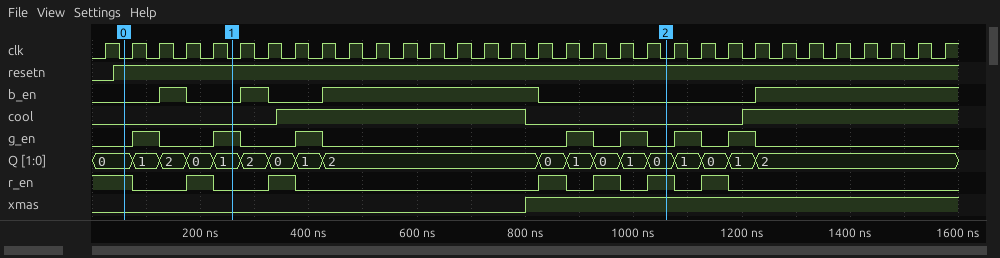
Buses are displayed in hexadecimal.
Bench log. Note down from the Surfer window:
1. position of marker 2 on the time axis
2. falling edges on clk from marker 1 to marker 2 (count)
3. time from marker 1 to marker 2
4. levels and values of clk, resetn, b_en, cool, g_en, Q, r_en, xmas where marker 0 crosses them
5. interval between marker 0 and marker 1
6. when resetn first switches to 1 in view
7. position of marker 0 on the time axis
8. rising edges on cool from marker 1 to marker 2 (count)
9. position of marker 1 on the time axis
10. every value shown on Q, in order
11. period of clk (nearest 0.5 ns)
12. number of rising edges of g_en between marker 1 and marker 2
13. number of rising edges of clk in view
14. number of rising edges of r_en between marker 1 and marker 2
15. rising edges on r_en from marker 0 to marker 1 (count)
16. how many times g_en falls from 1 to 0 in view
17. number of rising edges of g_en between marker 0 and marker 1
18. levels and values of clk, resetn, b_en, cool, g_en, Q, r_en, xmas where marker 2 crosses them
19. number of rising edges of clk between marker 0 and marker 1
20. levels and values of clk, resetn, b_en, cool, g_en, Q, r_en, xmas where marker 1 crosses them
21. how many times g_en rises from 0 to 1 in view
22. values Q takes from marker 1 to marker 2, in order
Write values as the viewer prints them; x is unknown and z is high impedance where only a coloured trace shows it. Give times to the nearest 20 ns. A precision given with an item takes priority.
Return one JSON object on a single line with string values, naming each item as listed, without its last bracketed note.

{"position of marker 2 on the time axis": "1060 ns", "falling edges on clk from marker 1 to marker 2": "16", "time from marker 1 to marker 2": "800 ns", "levels and values of clk, resetn, b_en, cool, g_en, Q, r_en, xmas where marker 0 crosses them": "clk=0, resetn=1, b_en=0, cool=0, g_en=0, Q=0, r_en=1, xmas=0", "interval between marker 0 and marker 1": "200 ns", "when resetn first switches to 1 in view": "40 ns", "position of marker 0 on the time axis": "60 ns", "rising edges on cool from marker 1 to marker 2": "1", "position of marker 1 on the time axis": "260 ns", "every value shown on Q, in order": "0, 1, 2, 0, 1, 2, 0, 1, 2, 0, 1, 0, 1, 0, 1, 0, 1, 2", "period of clk": "50 ns", "number of rising edges of g_en between marker 1 and marker 2": "3", "number of rising edges of clk in view": "32", "number of rising edges of r_en between marker 1 and marker 2": "4", "rising edges on r_en from marker 0 to marker 1": "1", "how many times g_en falls from 1 to 0 in view": "7", "number of rising edges of g_en between marker 0 and marker 1": "2", "levels and values of clk, resetn, b_en, cool, g_en, Q, r_en, xmas where marker 2 crosses them": "clk=0, resetn=1, b_en=0, cool=0, g_en=0, Q=0, r_en=1, xmas=1", "number of rising edges of clk between marker 0 and marker 1": "4", "levels and values of clk, resetn, b_en, cool, g_en, Q, r_en, xmas where marker 1 crosses them": "clk=0, resetn=1, b_en=0, cool=0, g_en=1, Q=1, r_en=0, xmas=0", "how many times g_en rises from 0 to 1 in view": "7", "values Q takes from marker 1 to marker 2, in order": "1, 2, 0, 1, 2, 0, 1, 0, 1, 0"}
